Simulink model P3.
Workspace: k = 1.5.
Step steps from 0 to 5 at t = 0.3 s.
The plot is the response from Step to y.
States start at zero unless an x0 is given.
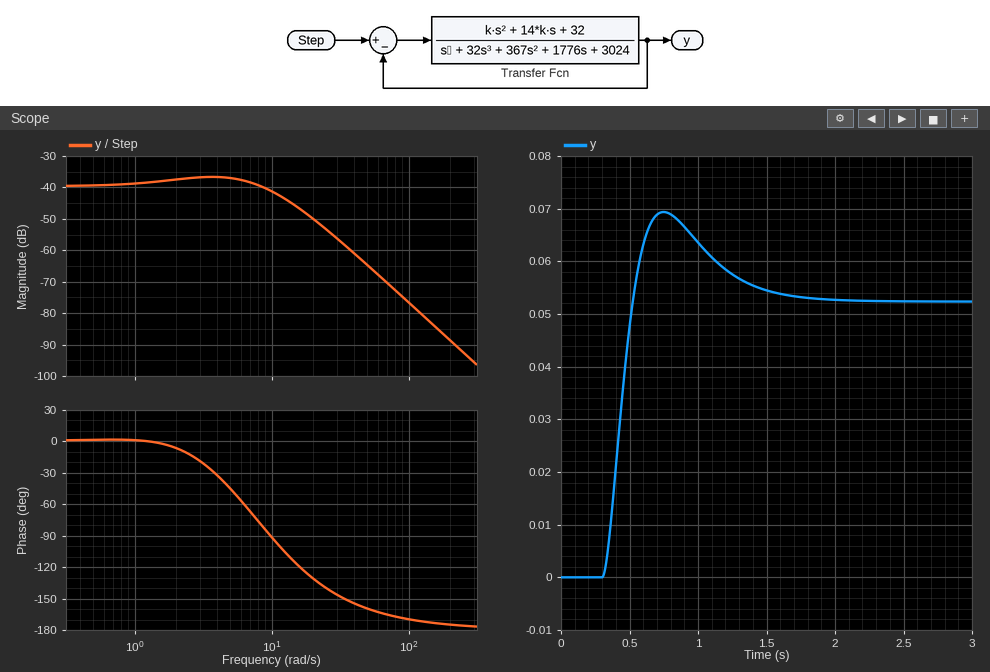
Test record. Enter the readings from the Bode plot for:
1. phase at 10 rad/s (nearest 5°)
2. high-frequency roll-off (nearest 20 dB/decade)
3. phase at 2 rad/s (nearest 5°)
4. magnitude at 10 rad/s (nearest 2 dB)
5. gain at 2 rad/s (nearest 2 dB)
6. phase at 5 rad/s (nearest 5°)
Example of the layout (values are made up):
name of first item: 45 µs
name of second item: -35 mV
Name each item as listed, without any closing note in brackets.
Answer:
phase at 10 rad/s: -90°
high-frequency roll-off: -40 dB/decade
phase at 2 rad/s: -5°
magnitude at 10 rad/s: -42 dB
gain at 2 rad/s: -38 dB
phase at 5 rad/s: -45°
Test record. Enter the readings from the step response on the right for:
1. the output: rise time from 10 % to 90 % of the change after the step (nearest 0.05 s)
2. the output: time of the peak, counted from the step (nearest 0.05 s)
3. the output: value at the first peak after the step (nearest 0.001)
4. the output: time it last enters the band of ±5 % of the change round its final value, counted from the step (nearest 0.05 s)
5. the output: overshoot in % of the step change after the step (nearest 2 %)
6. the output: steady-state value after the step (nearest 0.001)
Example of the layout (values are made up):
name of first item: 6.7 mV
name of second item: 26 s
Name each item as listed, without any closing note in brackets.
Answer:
the output: rise time from 10 % to 90 % of the change after the step: 0.15 s
the output: time of the peak, counted from the step: 0.45 s
the output: value at the first peak after the step: 0.069
the output: time it last enters the band of ±5 % of the change round its final value, counted from the step: 1.15 s
the output: overshoot in % of the step change after the step: 32 %
the output: steady-state value after the step: 0.052
